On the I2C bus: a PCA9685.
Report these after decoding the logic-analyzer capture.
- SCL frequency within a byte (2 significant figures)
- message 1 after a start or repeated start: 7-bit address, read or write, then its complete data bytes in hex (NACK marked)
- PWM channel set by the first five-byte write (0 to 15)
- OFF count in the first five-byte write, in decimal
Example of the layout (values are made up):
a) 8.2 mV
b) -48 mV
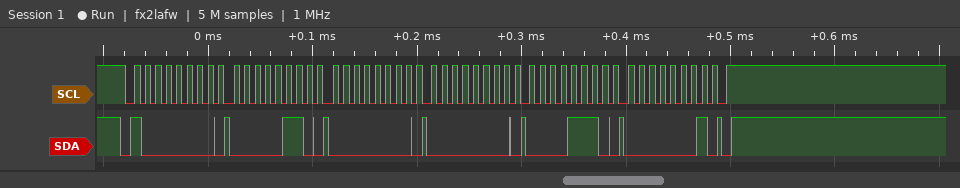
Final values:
a) 100 kHz
b) 0x40 write: 06 00 00 0E 01
c) 0
d) 270
